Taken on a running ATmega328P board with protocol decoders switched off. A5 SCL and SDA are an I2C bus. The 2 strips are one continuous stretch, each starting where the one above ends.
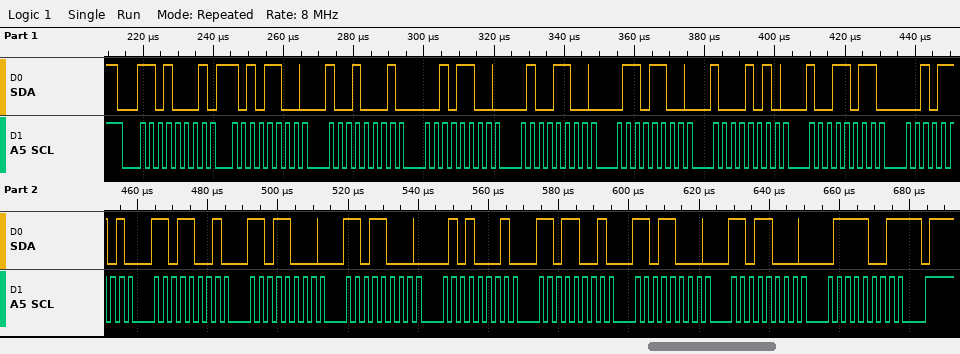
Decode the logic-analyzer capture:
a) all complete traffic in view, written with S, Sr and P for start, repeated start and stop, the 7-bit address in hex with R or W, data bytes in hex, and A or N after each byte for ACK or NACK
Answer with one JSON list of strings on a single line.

["S 68R A AC A 91 A 2C A 4C A 6C A 8A A 9B A 2D A D9 A D8 A D8 A 51 A D9 A D8 A D8 A 79 N P"]
